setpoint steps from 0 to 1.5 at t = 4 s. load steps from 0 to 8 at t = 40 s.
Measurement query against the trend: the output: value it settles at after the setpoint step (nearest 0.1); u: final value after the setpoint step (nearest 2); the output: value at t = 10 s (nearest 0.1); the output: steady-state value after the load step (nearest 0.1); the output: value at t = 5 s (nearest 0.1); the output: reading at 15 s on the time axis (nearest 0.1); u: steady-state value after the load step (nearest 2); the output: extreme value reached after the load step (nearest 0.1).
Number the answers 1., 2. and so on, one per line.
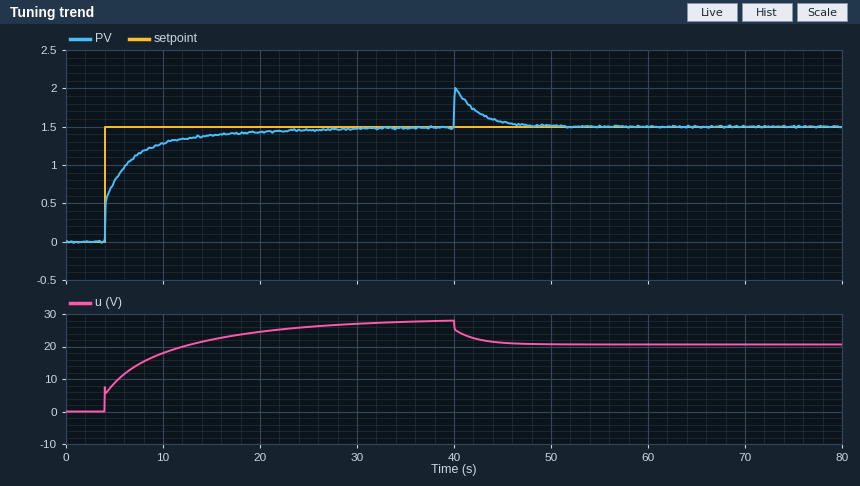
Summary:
1. 1.5
2. 28
3. 1.3
4. 1.5
5. 0.8
6. 1.4
7. 20
8. 2.0
